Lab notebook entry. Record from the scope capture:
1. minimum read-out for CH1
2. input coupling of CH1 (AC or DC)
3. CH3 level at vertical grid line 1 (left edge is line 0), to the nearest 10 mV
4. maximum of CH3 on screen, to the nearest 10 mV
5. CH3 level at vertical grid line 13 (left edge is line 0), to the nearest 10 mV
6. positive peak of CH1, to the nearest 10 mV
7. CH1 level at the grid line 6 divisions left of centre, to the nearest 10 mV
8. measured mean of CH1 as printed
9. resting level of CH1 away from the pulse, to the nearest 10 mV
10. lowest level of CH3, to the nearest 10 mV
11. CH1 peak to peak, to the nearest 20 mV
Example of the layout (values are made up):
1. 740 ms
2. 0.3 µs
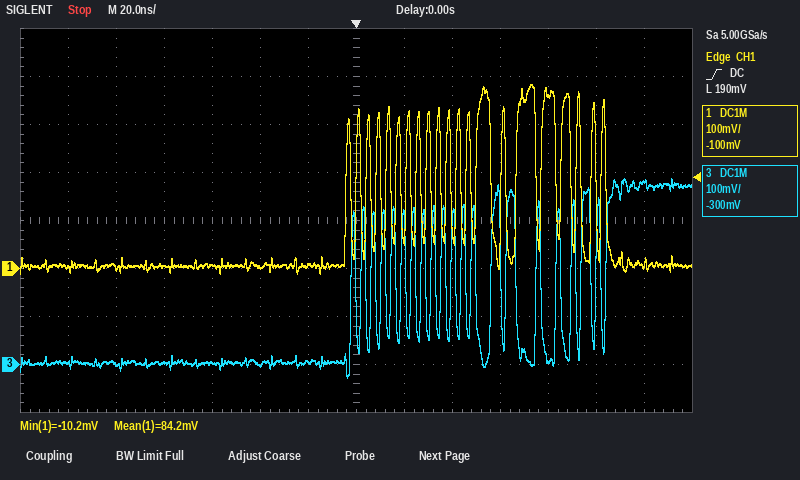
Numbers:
1. -10.2 mV
2. DC
3. 0 mV
4. 390 mV
5. 380 mV
6. 380 mV
7. 0 mV
8. 84.2 mV
9. 10 mV
10. -30 mV
11. 400 mV
